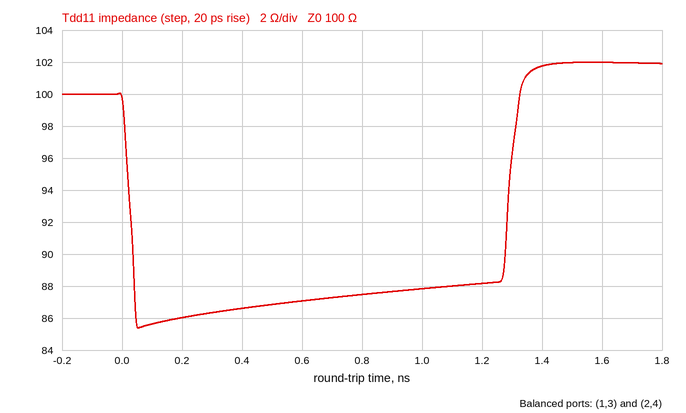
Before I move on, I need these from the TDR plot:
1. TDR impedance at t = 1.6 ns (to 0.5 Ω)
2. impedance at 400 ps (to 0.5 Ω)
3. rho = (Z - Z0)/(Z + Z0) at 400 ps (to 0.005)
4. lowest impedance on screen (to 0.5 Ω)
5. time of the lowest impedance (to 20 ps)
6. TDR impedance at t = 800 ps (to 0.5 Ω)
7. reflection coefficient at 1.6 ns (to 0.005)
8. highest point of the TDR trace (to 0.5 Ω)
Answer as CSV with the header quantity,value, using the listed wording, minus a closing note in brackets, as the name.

quantity,value
TDR impedance at t = 1.6 ns,102.0 Ω
impedance at 400 ps,86.5 Ω
rho = (Z - Z0)/(Z + Z0) at 400 ps,-0.070
lowest impedance on screen,85.5 Ω
time of the lowest impedance,60 ps
TDR impedance at t = 800 ps,87.5 Ω
reflection coefficient at 1.6 ns,+0.010
highest point of the TDR trace,102.0 Ω
